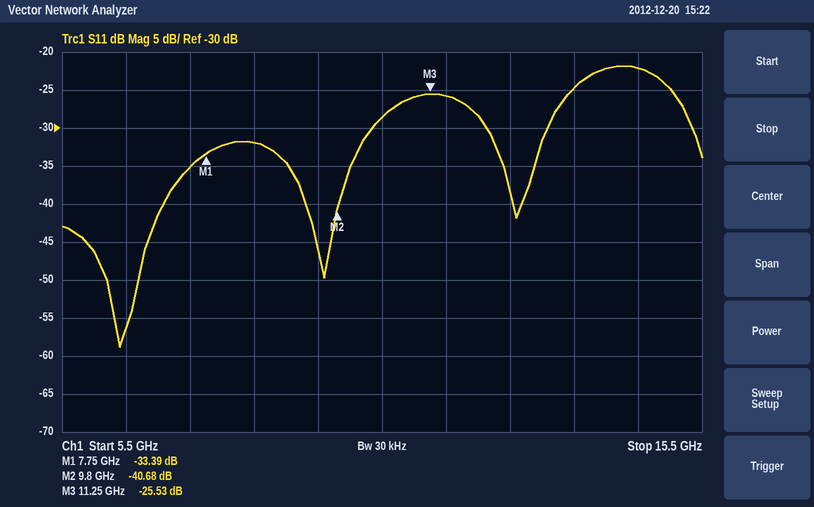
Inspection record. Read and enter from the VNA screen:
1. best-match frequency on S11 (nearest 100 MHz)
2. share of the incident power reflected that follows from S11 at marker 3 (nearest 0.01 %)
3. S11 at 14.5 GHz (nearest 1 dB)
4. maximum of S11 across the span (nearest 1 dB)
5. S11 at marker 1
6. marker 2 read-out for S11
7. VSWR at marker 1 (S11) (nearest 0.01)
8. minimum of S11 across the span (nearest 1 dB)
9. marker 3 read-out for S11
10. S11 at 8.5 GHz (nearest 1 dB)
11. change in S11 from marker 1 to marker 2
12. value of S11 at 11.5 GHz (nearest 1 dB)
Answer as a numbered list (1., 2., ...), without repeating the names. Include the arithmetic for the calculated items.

1. 6.4 GHz
2. 10^(-25.53/10) ≈ 0.28 %
3. -22 dB
4. -22 dB
5. -33.39 dB
6. -40.68 dB
7. (1 + 0.0214)/(1 − 0.0214) ≈ 1.04
8. -59 dB
9. -25.53 dB
10. -32 dB
11. -40.68 − (-33.39) = -7.29 dB
12. -26 dB
